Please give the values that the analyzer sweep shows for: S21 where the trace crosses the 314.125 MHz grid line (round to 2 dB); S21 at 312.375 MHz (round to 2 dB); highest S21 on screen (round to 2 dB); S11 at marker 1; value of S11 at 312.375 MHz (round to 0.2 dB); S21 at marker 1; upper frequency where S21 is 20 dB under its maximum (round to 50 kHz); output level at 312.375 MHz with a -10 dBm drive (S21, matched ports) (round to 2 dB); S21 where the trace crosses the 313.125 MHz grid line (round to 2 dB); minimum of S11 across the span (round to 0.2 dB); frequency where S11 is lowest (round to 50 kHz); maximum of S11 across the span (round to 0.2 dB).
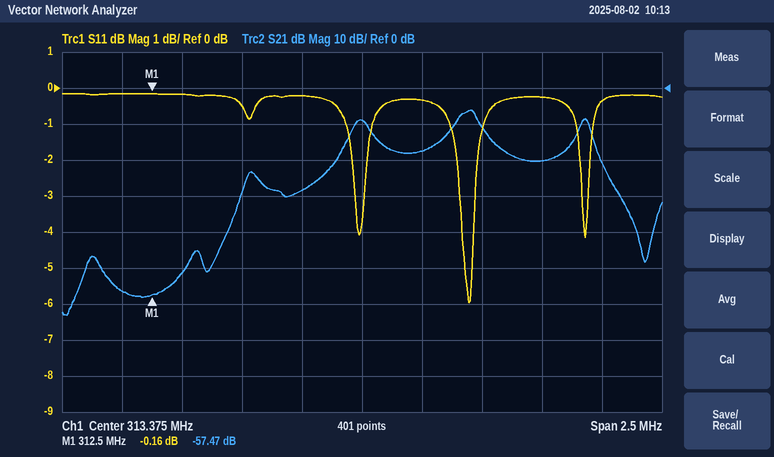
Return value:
-20 dB
-56 dB
-6 dB
-0.16 dB
-0.2 dB
-57.47 dB
314.40 MHz
-66 dBm
-28 dB
-6.0 dB
313.80 MHz
-0.2 dB
